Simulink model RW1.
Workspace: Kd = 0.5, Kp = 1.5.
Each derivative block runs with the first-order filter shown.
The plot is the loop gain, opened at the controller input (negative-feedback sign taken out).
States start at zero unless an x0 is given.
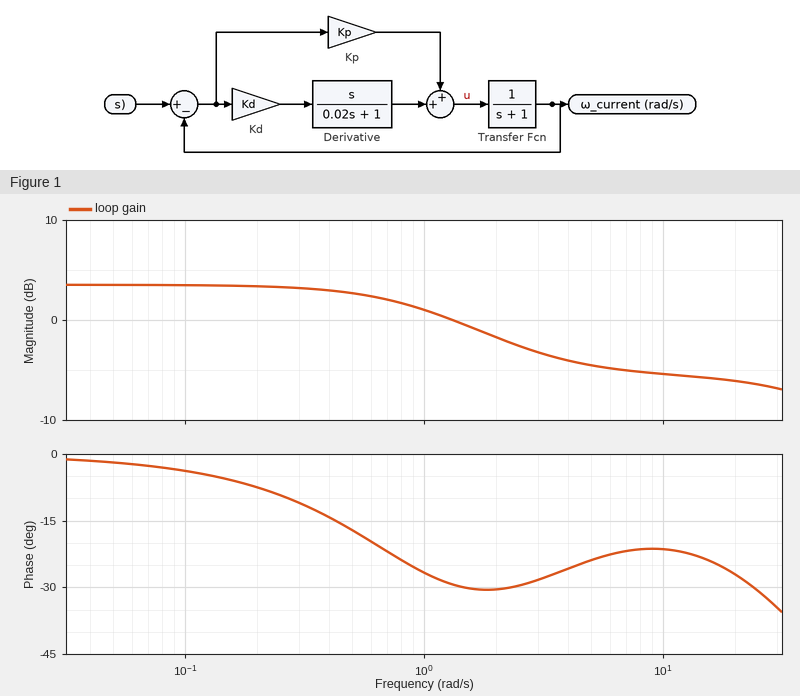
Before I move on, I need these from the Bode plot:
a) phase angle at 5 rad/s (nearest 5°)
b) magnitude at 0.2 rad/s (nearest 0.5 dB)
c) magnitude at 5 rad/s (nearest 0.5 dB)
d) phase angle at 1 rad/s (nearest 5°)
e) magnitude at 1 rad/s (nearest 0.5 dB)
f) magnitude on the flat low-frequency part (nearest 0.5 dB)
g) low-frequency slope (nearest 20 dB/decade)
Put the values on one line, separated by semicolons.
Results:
-25°; 3.5 dB; -4.5 dB; -25°; 1.0 dB; 3.5 dB; 0 dB/decade
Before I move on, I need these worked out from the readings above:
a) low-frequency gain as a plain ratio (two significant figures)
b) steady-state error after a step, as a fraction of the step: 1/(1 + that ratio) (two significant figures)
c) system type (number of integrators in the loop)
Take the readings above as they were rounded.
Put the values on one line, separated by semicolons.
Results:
1.5; 0.40; 0
